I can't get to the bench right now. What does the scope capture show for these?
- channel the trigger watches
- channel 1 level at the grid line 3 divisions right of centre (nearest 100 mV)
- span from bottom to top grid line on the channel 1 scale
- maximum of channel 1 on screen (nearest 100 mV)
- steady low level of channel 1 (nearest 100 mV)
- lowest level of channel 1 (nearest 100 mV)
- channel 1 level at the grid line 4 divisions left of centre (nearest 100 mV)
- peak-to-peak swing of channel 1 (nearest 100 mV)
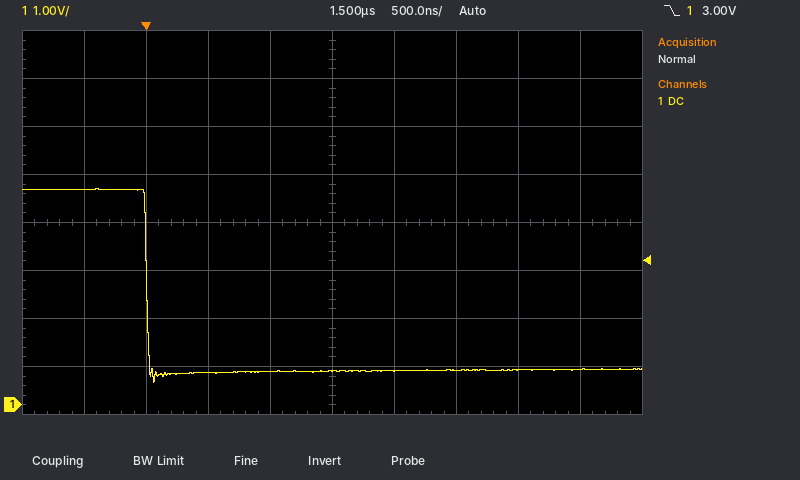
channel 1
700 mV
8 V
4.5 V
700 mV
500 mV
4.5 V
4.0 V
